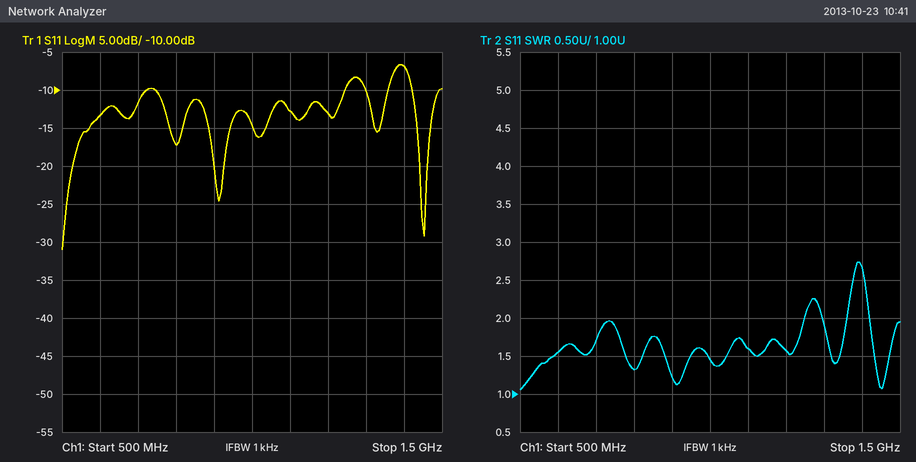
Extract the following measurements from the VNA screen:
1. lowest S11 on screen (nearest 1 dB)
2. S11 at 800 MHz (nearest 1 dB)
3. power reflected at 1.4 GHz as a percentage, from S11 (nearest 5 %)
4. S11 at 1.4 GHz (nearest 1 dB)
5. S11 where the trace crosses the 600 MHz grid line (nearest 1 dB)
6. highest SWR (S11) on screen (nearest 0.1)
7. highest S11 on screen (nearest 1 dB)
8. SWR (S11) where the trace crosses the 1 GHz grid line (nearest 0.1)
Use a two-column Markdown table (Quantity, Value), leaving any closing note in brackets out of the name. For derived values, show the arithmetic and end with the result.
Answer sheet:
| Quantity | Value |
|---|---|
| lowest S11 on screen | -31 dB |
| S11 at 800 MHz | -17 dB |
| power reflected at 1.4 GHz as a percentage, from S11 | 10^(-7/10) ≈ 20 % |
| S11 at 1.4 GHz | -7 dB |
| S11 where the trace crosses the 600 MHz grid line | -13 dB |
| highest SWR (S11) on screen | 2.7 |
| highest S11 on screen | -7 dB |
| SWR (S11) where the trace crosses the 1 GHz grid line | 1.5 |
